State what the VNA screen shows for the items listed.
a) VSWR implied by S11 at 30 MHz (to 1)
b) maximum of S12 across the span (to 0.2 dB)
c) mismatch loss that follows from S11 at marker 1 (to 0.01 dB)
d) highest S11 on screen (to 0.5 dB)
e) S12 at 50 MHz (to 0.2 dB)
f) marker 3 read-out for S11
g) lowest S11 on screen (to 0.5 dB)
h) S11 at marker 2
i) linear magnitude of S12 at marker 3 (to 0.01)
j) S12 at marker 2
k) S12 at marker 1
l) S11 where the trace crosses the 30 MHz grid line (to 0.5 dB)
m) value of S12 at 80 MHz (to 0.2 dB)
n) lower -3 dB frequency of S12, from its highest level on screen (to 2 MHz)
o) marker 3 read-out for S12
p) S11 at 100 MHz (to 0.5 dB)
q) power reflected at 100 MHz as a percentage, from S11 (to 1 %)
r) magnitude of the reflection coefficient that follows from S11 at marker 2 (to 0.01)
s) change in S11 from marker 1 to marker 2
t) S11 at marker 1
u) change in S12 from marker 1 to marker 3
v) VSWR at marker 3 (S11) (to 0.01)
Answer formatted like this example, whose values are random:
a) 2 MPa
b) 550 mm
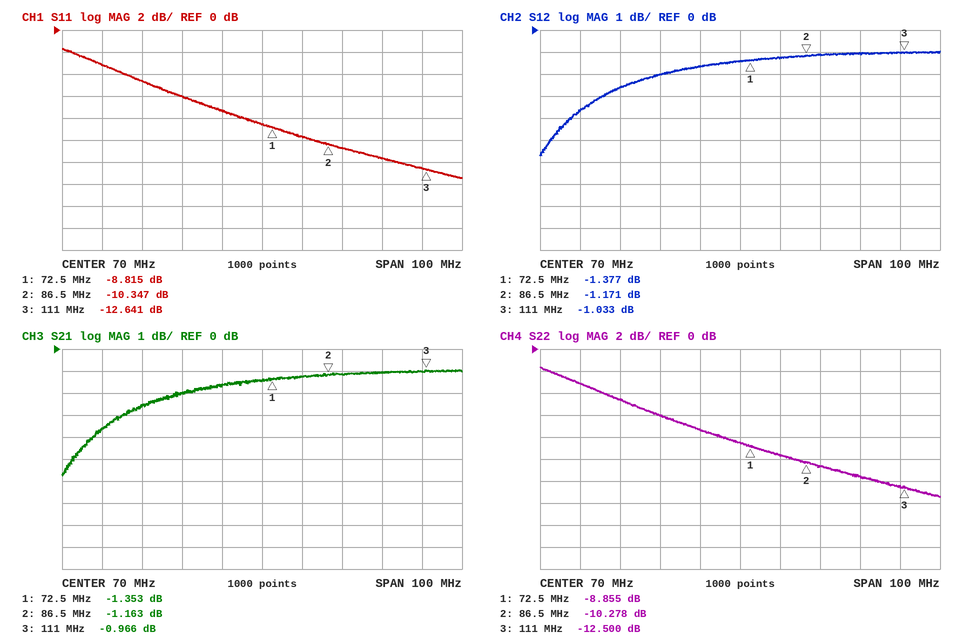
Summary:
a) 6
b) -1.0 dB
c) 0.61 dB
d) -1.5 dB
e) -2.0 dB
f) -12.641 dB
g) -13.5 dB
h) -10.347 dB
i) 0.89
j) -1.171 dB
k) -1.377 dB
l) -3.0 dB
m) -1.2 dB
n) 28 MHz
o) -1.033 dB
p) -11.5 dB
q) 7 %
r) 0.30
s) -1.532 dB
t) -8.815 dB
u) 0.344 dB
v) 1.61
